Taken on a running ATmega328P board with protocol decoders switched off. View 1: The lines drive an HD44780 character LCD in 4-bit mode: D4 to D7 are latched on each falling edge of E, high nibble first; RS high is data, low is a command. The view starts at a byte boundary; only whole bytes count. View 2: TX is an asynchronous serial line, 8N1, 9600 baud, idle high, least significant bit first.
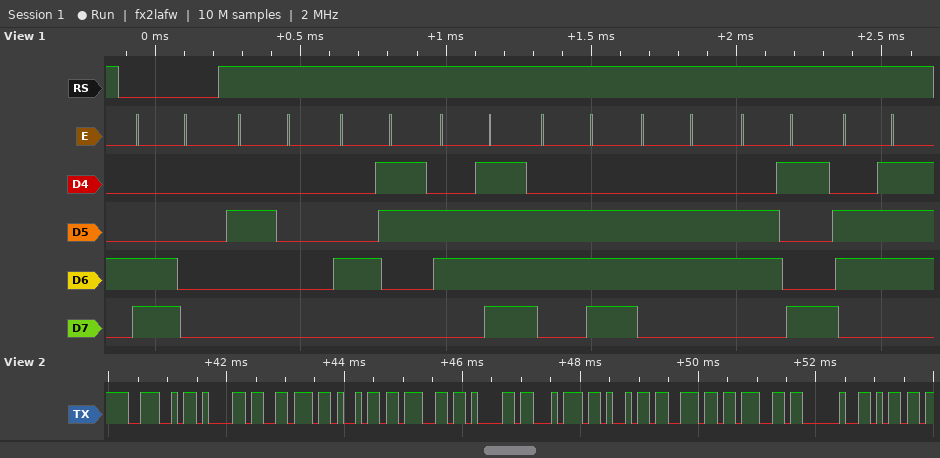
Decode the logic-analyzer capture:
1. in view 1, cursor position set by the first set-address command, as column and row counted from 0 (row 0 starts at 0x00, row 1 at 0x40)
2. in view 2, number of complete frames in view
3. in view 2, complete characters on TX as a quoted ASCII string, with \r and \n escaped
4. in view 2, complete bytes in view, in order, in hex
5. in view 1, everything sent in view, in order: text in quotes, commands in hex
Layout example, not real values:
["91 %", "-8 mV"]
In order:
["column 0, row 1", "12", "\"Navigating m\"", "4E 61 76 69 67 61 74 69 6E 67 20 6D", "0xC0 \" Config\""]
